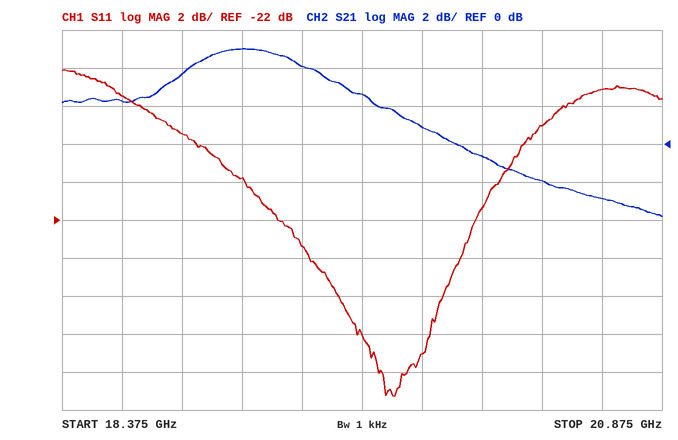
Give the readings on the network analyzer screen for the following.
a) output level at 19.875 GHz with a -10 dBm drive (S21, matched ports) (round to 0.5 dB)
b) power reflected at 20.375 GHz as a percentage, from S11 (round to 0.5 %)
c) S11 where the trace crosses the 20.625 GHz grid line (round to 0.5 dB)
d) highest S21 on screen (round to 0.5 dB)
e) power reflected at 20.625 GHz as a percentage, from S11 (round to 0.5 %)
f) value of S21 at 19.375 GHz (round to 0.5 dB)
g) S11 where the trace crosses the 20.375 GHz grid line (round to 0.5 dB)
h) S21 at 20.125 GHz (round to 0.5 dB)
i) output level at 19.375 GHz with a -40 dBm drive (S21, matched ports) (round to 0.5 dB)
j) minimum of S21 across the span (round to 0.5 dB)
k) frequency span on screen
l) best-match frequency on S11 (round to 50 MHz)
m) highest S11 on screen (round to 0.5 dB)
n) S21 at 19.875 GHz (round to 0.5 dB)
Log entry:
-9.0 dBm
2.0 %
-15.0 dB
5.0 dB
3.0 %
4.0 dB
-17.0 dB
-0.5 dB
-36.0 dBm
-4.0 dB
2.5 GHz
19.75 GHz
-14.0 dB
1.0 dB
